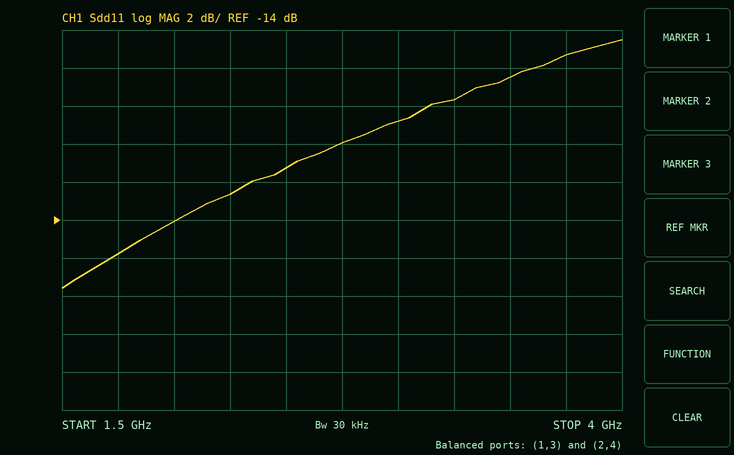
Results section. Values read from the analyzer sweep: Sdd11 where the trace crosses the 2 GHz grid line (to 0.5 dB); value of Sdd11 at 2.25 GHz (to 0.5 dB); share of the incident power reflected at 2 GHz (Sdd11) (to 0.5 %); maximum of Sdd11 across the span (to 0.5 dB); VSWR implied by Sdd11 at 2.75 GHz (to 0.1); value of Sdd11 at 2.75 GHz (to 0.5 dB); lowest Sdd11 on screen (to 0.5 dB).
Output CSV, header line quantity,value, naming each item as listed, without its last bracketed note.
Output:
quantity,value
Sdd11 where the trace crosses the 2 GHz grid line,-14.0 dB
value of Sdd11 at 2.25 GHz,-12.5 dB
share of the incident power reflected at 2 GHz (Sdd11),4.0 %
maximum of Sdd11 across the span,-4.5 dB
VSWR implied by Sdd11 at 2.75 GHz,1.9
value of Sdd11 at 2.75 GHz,-10.0 dB
lowest Sdd11 on screen,-17.5 dB
